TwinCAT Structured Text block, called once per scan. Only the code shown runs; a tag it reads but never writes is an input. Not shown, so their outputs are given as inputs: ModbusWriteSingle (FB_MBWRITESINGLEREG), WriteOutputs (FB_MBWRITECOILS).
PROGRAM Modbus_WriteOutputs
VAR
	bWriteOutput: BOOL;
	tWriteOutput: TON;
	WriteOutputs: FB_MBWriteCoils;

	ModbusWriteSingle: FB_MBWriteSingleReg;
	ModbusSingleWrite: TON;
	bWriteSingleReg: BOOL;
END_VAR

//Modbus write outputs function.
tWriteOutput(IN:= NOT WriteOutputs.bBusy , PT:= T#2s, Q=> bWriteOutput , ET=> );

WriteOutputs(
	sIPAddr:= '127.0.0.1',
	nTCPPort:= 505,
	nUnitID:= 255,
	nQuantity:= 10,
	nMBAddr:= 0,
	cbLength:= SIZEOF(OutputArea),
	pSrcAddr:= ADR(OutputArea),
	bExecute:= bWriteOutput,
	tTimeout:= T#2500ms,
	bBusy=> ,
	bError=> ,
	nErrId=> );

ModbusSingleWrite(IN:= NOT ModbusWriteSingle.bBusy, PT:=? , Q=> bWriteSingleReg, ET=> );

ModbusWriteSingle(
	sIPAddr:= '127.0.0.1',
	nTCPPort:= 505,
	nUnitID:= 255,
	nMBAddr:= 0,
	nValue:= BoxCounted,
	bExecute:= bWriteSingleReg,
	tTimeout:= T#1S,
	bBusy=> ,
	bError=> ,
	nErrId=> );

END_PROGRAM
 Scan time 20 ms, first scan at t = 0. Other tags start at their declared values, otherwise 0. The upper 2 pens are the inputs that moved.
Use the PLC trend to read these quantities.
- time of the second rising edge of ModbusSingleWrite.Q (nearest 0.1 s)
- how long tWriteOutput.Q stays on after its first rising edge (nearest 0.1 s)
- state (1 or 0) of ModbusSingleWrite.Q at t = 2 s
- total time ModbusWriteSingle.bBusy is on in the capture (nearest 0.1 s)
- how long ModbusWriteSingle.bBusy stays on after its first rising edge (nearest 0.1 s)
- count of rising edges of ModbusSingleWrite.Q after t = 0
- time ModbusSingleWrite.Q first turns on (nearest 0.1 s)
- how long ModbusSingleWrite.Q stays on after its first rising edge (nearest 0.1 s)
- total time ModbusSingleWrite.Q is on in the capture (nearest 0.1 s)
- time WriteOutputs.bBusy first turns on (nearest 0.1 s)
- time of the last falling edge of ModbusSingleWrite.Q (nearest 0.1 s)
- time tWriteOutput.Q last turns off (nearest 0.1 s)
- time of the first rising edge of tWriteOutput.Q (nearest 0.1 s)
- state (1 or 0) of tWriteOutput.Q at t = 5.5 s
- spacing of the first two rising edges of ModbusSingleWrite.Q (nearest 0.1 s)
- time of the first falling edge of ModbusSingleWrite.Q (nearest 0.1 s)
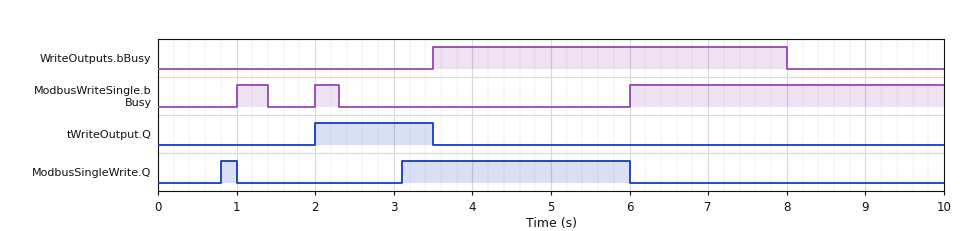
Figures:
3.1 s
1.5 s
0
4.7 s
0.4 s
2
0.8 s
0.2 s
3.1 s
3.5 s
6.0 s
3.5 s
2.0 s
0
2.3 s
1.0 s
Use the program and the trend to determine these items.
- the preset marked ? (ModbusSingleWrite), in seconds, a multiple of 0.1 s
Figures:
0.8 s
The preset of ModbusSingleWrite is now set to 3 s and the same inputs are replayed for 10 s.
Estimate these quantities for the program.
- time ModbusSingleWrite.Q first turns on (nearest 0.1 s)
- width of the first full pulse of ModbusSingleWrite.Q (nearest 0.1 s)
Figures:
5.3 s
0.7 s
